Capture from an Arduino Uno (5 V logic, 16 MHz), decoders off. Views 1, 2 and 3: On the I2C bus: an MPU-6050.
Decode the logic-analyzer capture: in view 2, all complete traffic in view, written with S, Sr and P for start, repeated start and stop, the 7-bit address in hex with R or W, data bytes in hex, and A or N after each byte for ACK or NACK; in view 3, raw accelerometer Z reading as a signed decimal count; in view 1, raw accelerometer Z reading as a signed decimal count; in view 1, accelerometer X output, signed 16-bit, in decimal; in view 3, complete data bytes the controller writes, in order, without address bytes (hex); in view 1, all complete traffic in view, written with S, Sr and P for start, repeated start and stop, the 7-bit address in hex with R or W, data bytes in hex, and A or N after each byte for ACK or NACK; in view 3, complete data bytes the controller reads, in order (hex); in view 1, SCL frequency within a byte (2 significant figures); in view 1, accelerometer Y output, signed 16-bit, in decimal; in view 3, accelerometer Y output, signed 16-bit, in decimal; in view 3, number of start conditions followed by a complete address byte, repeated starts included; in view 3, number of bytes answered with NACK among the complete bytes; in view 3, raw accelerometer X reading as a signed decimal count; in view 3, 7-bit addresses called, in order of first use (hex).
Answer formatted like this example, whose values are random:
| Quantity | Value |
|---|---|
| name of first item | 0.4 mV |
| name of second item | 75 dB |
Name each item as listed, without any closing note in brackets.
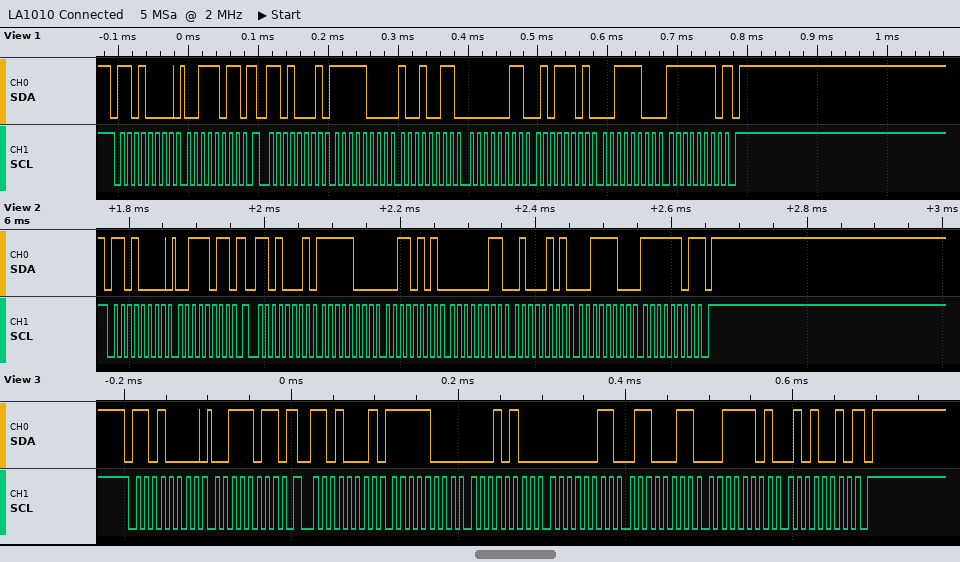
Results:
| Quantity | Value |
|---|---|
| in view 2, all complete traffic in view, written with S, Sr and P for start, repeated start and stop, the 7-bit address in hex with R or W, data bytes in hex, and A or N after each byte for ACK or NACK | S 68W A 3B A Sr 68R A F8 A 35 A 03 A 45 A 3C A FD N P |
| in view 3, raw accelerometer Z reading as a signed decimal count | 15698 |
| in view 1, raw accelerometer Z reading as a signed decimal count | 15614 |
| in view 1, accelerometer X output, signed 16-bit, in decimal | -1901 |
| in view 3, complete data bytes the controller writes, in order, without address bytes | 3B |
| in view 1, all complete traffic in view, written with S, Sr and P for start, repeated start and stop, the 7-bit address in hex with R or W, data bytes in hex, and A or N after each byte for ACK or NACK | S 68W A 3B A Sr 68R A F8 A 93 A 03 A 5D A 3C A FE N P |
| in view 3, complete data bytes the controller reads, in order | F8 14 03 63 3D 52 |
| in view 1, SCL frequency within a byte | 100 kHz |
| in view 1, accelerometer Y output, signed 16-bit, in decimal | 861 |
| in view 3, accelerometer Y output, signed 16-bit, in decimal | 867 |
| in view 3, number of start conditions followed by a complete address byte, repeated starts included | 2 |
| in view 3, number of bytes answered with NACK among the complete bytes | 1 |
| in view 3, raw accelerometer X reading as a signed decimal count | -2028 |
| in view 3, 7-bit addresses called, in order of first use | 0x68 |
